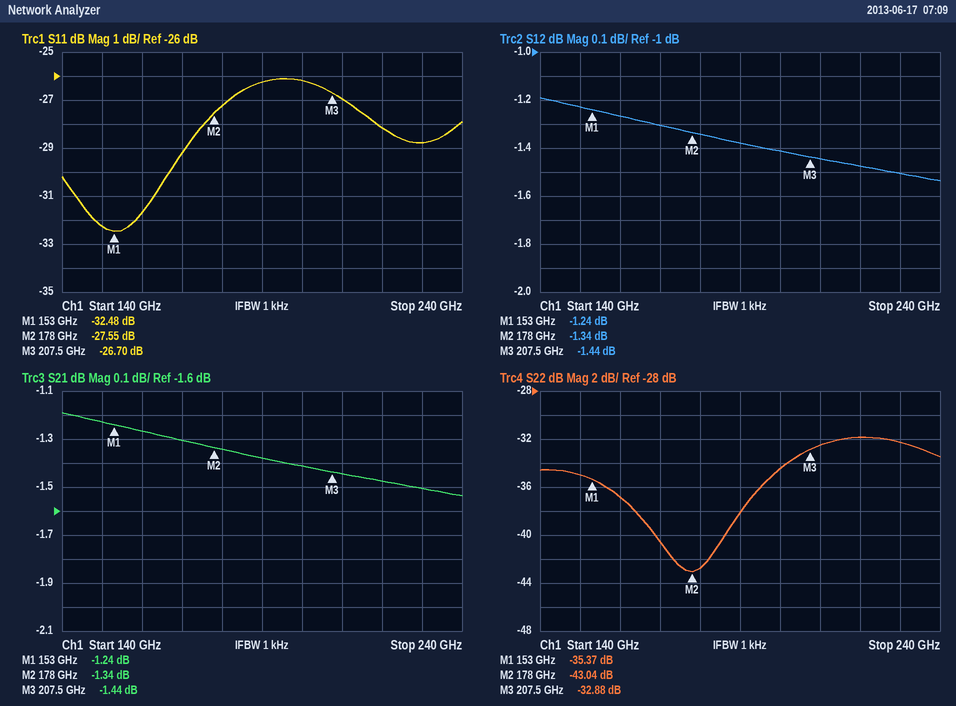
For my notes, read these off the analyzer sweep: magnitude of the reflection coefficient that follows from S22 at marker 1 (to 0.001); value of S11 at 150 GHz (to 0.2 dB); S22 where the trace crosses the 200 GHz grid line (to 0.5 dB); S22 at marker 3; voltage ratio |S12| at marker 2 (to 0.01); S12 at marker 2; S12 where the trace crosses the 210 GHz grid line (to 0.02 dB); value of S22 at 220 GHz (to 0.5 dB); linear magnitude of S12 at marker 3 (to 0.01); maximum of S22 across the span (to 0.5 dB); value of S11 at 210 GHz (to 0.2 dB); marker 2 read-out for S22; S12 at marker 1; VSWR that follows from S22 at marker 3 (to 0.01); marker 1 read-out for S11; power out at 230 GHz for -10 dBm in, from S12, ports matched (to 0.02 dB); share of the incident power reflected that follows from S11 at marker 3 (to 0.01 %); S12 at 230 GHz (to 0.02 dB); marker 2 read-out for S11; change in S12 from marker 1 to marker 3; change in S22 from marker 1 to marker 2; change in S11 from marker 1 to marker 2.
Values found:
0.017
-32.2 dB
-34.5 dB
-32.88 dB
0.86
-1.34 dB
-1.44 dB
-32.0 dB
0.85
-32.0 dB
-27.0 dB
-43.04 dB
-1.24 dB
1.05
-32.48 dB
-11.50 dBm
0.21 %
-1.50 dB
-27.55 dB
-0.20 dB
-7.67 dB
4.93 dB
